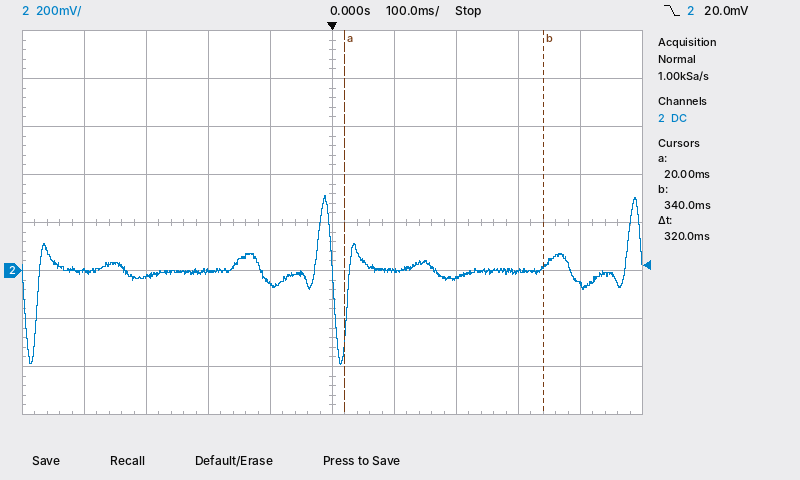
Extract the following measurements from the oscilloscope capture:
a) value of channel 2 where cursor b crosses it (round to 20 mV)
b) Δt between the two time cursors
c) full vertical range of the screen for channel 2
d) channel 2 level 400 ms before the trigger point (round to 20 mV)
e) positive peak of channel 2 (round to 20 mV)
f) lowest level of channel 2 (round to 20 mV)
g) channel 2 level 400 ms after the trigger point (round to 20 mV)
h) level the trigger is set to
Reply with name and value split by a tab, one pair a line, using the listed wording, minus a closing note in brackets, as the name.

value of channel 2 where cursor b crosses it	20 mV
Δt between the two time cursors	320 ms
full vertical range of the screen for channel 2	1.6 V
channel 2 level 400 ms before the trigger point	0 mV
positive peak of channel 2	320 mV
lowest level of channel 2	-400 mV
channel 2 level 400 ms after the trigger point	-60 mV
level the trigger is set to	20.0 mV
